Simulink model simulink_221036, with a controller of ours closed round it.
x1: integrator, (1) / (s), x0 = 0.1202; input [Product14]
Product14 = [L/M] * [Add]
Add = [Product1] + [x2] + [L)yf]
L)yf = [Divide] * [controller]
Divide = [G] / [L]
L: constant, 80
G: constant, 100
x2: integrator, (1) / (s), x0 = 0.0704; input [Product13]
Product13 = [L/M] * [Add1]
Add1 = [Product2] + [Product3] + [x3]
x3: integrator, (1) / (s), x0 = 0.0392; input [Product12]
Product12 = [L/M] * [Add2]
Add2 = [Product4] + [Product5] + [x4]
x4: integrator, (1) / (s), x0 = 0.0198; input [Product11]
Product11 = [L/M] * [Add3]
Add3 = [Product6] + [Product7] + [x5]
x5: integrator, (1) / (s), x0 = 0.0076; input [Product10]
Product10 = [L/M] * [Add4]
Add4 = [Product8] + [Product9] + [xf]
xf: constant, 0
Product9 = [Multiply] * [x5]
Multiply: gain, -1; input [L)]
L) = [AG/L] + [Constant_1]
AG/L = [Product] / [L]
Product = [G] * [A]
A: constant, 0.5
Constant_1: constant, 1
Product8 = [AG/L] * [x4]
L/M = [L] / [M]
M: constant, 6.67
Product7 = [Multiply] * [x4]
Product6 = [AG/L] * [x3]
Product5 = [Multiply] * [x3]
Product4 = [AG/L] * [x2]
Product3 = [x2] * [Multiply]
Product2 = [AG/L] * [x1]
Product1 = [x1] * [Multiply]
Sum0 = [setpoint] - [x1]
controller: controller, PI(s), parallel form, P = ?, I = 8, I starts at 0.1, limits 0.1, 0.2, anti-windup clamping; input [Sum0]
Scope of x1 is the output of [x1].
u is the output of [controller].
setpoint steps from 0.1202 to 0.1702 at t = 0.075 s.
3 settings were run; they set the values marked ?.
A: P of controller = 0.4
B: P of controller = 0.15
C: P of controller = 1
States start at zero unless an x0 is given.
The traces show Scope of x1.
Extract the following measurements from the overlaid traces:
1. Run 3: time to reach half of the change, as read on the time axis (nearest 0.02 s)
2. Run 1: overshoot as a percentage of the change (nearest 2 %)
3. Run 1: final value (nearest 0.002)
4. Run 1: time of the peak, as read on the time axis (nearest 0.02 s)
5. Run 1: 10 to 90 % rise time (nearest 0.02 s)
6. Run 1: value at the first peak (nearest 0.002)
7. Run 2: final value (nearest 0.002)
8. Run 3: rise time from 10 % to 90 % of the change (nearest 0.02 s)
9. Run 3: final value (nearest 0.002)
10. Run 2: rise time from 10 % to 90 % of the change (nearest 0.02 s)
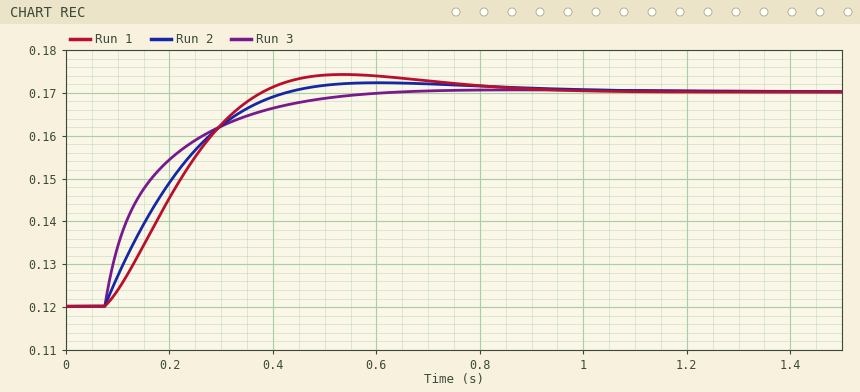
0.14 s
8 %
0.170
0.54 s
0.22 s
0.174
0.170
0.28 s
0.170
0.24 s
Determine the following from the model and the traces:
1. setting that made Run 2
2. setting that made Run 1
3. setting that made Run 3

A
B
C
